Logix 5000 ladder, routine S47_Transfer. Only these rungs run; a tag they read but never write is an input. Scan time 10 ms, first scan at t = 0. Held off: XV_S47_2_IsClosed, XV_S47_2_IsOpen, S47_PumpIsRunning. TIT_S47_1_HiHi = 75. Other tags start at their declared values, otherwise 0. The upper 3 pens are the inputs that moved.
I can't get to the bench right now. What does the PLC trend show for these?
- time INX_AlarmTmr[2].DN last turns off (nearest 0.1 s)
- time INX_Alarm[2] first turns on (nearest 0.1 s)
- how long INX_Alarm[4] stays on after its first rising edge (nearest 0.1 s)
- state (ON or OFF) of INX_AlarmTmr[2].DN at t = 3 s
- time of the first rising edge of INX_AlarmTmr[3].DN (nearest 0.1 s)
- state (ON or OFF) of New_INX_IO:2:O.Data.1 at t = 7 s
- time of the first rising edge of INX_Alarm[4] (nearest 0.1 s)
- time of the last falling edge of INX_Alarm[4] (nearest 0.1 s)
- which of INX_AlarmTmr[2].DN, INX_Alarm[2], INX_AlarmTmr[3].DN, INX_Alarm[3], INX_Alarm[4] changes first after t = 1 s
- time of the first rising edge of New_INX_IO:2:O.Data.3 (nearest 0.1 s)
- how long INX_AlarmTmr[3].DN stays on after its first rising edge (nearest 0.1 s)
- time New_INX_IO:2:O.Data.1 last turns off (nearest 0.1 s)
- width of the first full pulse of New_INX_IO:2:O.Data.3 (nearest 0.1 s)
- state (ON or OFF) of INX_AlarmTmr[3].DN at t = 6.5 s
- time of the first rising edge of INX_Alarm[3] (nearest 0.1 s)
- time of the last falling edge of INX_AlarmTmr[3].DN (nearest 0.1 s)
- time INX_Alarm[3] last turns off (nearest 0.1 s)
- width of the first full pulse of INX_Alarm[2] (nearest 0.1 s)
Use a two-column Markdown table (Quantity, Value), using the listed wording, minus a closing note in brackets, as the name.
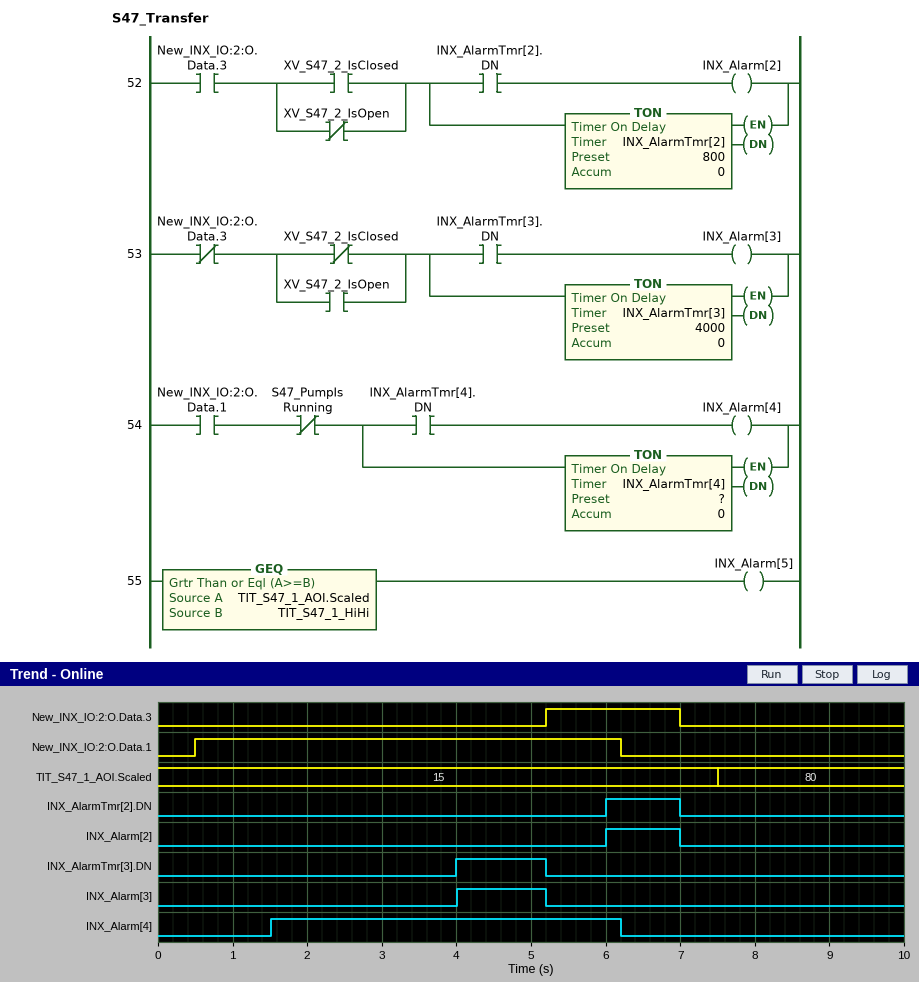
| Quantity | Value |
|---|---|
| time INX_AlarmTmr[2].DN last turns off | 7.0 s |
| time INX_Alarm[2] first turns on | 6.0 s |
| how long INX_Alarm[4] stays on after its first rising edge | 4.7 s |
| state (ON or OFF) of INX_AlarmTmr[2].DN at t = 3 s | OFF |
| time of the first rising edge of INX_AlarmTmr[3].DN | 4.0 s |
| state (ON or OFF) of New_INX_IO:2:O.Data.1 at t = 7 s | OFF |
| time of the first rising edge of INX_Alarm[4] | 1.5 s |
| time of the last falling edge of INX_Alarm[4] | 6.2 s |
| which of INX_AlarmTmr[2].DN, INX_Alarm[2], INX_AlarmTmr[3].DN, INX_Alarm[3], INX_Alarm[4] changes first after t = 1 s | INX_Alarm[4] |
| time of the first rising edge of New_INX_IO:2:O.Data.3 | 5.2 s |
| how long INX_AlarmTmr[3].DN stays on after its first rising edge | 1.2 s |
| time New_INX_IO:2:O.Data.1 last turns off | 6.2 s |
| width of the first full pulse of New_INX_IO:2:O.Data.3 | 1.8 s |
| state (ON or OFF) of INX_AlarmTmr[3].DN at t = 6.5 s | OFF |
| time of the first rising edge of INX_Alarm[3] | 4.0 s |
| time of the last falling edge of INX_AlarmTmr[3].DN | 5.2 s |
| time INX_Alarm[3] last turns off | 5.2 s |
| width of the first full pulse of INX_Alarm[2] | 1.0 s |
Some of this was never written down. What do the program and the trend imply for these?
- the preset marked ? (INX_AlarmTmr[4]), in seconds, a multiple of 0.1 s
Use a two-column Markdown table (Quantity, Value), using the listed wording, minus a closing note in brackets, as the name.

| Quantity | Value |
|---|---|
| the preset marked ? (INX_AlarmTmr[4]), in seconds, a multiple of 0.1 s | 1.0 s |
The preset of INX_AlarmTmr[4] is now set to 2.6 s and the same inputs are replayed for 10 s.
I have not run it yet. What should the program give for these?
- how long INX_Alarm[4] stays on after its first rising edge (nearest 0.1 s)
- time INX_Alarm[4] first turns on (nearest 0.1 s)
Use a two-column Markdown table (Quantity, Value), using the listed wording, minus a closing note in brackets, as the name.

| Quantity | Value |
|---|---|
| how long INX_Alarm[4] stays on after its first rising edge | 3.1 s |
| time INX_Alarm[4] first turns on | 3.1 s |
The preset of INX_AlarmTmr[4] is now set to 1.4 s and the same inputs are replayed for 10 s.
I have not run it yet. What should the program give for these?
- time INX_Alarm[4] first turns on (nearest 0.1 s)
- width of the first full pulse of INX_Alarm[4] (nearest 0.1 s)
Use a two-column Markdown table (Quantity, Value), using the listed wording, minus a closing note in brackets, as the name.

| Quantity | Value |
|---|---|
| time INX_Alarm[4] first turns on | 1.9 s |
| width of the first full pulse of INX_Alarm[4] | 4.3 s |
